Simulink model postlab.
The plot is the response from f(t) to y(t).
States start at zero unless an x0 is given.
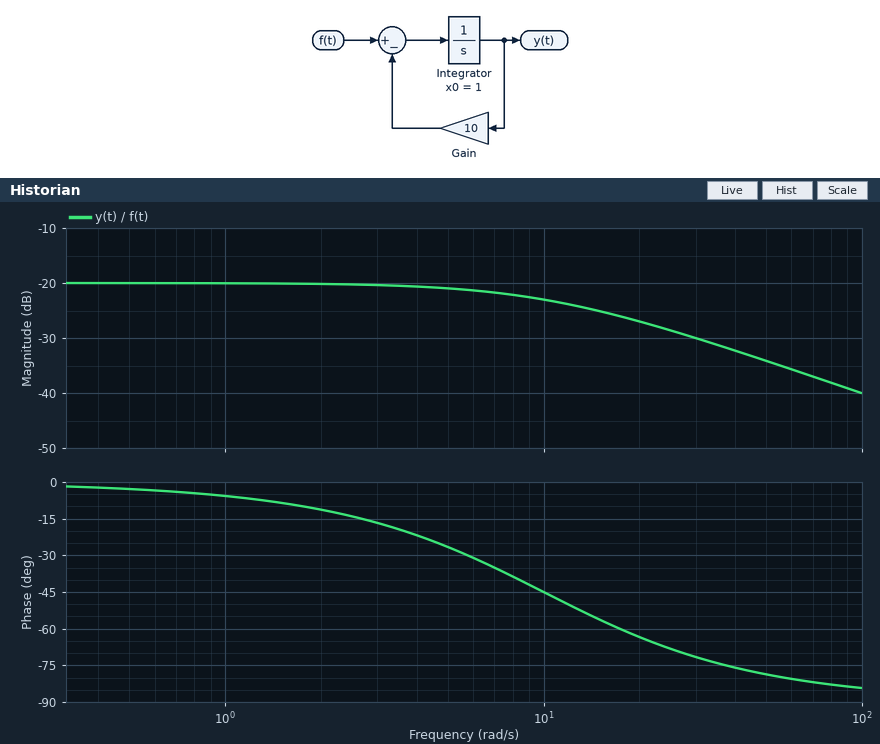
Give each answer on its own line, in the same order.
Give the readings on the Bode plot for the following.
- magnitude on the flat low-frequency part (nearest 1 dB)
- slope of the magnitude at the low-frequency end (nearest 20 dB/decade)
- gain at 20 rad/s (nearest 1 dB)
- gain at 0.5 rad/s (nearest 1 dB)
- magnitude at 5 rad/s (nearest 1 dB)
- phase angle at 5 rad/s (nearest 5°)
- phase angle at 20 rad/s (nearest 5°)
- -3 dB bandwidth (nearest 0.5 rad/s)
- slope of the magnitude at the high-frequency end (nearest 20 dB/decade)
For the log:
-20 dB
0 dB/decade
-27 dB
-20 dB
-21 dB
-25°
-65°
10.0 rad/s
-20 dB/decade
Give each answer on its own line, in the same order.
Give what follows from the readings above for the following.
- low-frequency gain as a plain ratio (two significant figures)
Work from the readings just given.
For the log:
0.10
